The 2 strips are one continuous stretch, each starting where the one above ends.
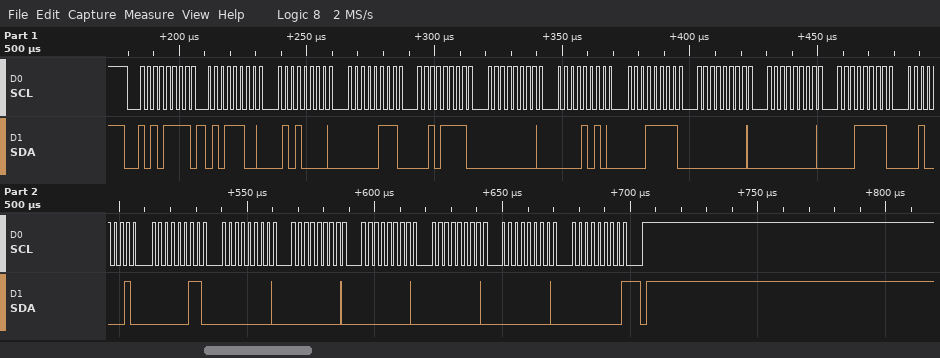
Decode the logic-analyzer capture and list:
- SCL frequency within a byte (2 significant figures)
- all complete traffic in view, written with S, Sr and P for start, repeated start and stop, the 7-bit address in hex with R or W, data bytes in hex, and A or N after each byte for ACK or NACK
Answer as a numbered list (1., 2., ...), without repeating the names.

1. 400 kHz
2. S 57R A 5C A 50 A 07 A 2F A 00 A 0A A 1F A 00 A 00 A 1F A 21 A 03 A 00 A 00 A 00 A 00 A 00 A 00 N P
